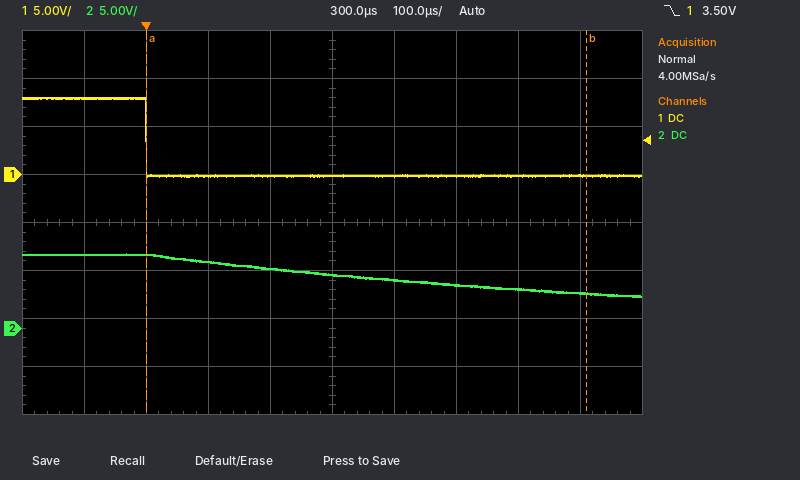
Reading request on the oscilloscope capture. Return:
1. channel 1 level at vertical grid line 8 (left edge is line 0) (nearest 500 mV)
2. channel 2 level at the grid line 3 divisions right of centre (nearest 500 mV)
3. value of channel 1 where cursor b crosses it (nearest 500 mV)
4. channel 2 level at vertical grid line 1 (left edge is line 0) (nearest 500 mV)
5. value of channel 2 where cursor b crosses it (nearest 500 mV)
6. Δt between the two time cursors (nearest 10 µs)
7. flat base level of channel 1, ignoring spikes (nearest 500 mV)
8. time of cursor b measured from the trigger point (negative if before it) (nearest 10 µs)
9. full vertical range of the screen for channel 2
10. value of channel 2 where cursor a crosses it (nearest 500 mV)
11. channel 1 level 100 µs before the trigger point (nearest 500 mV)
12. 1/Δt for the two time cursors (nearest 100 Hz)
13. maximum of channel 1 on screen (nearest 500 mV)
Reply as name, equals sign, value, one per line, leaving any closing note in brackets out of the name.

channel 1 level at vertical grid line 8 (left edge is line 0) = 0.0 V
channel 2 level at the grid line 3 divisions right of centre = 4.0 V
value of channel 1 where cursor b crosses it = 0.0 V
channel 2 level at vertical grid line 1 (left edge is line 0) = 7.5 V
value of channel 2 where cursor b crosses it = 3.5 V
Δt between the two time cursors = 710 µs
flat base level of channel 1, ignoring spikes = 0.0 V
time of cursor b measured from the trigger point (negative if before it) = +710 µs
full vertical range of the screen for channel 2 = 40 V
value of channel 2 where cursor a crosses it = 7.5 V
channel 1 level 100 µs before the trigger point = 8.0 V
1/Δt for the two time cursors = 1.4 kHz
maximum of channel 1 on screen = 8.0 V
